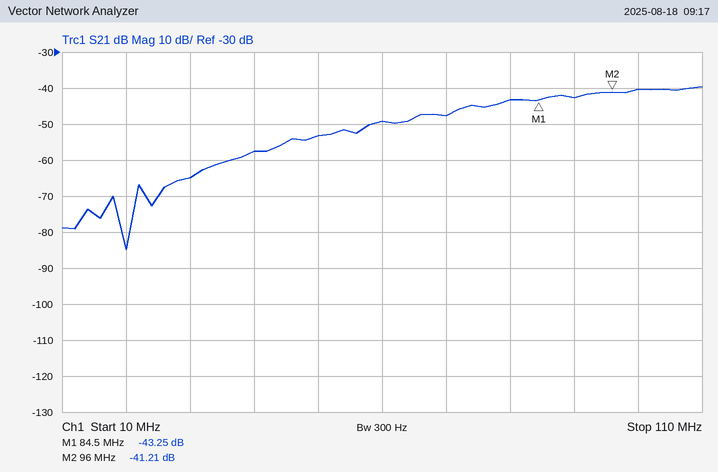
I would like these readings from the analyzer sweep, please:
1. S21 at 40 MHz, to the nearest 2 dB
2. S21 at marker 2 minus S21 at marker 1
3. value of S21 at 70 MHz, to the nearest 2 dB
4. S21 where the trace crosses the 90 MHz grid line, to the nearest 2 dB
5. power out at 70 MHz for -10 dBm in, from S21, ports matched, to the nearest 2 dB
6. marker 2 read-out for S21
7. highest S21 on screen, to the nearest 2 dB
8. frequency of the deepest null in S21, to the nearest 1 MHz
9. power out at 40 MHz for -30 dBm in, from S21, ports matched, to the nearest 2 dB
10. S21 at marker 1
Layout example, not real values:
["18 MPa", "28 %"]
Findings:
["-58 dB", "2.04 dB", "-48 dB", "-42 dB", "-58 dBm", "-41.21 dB", "-40 dB", "20 MHz", "-88 dBm", "-43.25 dB"]
